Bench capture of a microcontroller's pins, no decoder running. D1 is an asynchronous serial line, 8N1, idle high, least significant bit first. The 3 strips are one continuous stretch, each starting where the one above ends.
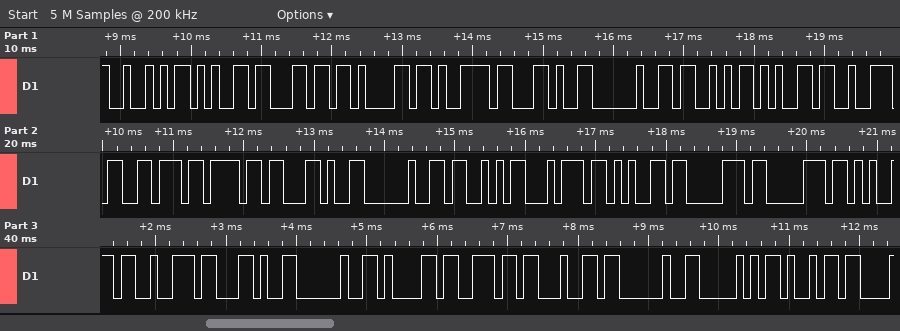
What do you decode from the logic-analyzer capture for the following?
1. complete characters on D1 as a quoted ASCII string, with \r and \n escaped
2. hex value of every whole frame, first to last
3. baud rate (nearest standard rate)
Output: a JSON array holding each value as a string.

["\"Relay, Servo, Stepper, and Pi\"", "52 65 6C 61 79 2C 20 53 65 72 76 6F 2C 20 53 74 65 70 70 65 72 2C 20 61 6E 64 20 50 69", "9600 baud"]
